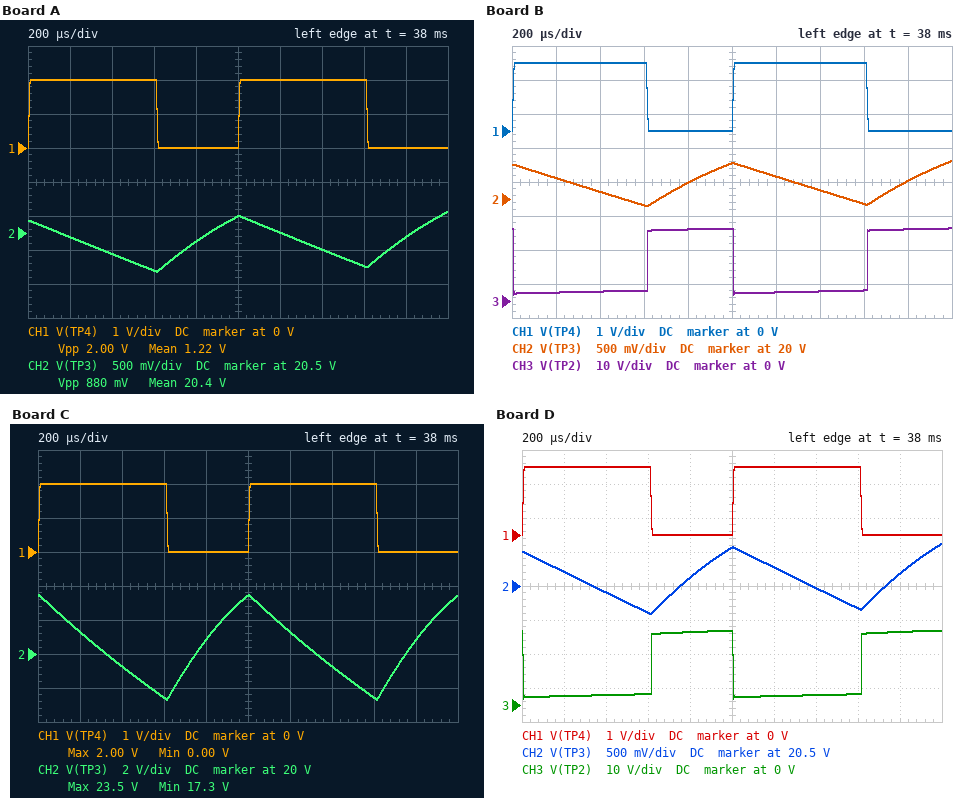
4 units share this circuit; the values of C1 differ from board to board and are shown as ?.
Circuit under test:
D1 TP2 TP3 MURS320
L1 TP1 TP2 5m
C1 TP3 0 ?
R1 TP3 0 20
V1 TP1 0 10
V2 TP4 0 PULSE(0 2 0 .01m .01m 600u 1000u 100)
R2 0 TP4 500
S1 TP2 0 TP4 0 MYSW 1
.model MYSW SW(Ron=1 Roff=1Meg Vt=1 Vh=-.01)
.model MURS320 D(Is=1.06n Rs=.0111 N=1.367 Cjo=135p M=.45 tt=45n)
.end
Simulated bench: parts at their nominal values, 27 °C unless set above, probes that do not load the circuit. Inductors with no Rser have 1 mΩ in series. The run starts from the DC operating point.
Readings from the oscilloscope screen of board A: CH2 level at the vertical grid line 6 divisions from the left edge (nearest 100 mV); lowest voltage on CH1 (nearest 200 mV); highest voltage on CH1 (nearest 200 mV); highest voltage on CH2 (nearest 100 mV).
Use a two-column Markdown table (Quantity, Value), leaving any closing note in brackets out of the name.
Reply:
| Quantity | Value |
|---|---|
| CH2 level at the vertical grid line 6 divisions from the left edge | 20.5 V |
| lowest voltage on CH1 | 0 V |
| highest voltage on CH1 | 2.0 V |
| highest voltage on CH2 | 20.8 V |
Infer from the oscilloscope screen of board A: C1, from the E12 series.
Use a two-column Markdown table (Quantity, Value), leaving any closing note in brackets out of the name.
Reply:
| Quantity | Value |
|---|---|
| C1, from the E12 series | 820 µF |
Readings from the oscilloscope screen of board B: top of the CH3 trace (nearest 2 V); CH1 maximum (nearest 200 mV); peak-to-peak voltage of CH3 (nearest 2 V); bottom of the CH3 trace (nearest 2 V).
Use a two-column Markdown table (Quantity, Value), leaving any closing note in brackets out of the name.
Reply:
| Quantity | Value |
|---|---|
| top of the CH3 trace | 22 V |
| CH1 maximum | 2.0 V |
| peak-to-peak voltage of CH3 | 20 V |
| bottom of the CH3 trace | 2 V |
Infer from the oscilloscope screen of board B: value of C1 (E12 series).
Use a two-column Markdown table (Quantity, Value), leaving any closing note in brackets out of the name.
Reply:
| Quantity | Value |
|---|---|
| value of C1 | 1 mF |
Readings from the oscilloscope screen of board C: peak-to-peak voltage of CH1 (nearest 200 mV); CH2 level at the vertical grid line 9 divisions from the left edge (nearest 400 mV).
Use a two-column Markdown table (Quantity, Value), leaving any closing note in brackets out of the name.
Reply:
| Quantity | Value |
|---|---|
| peak-to-peak voltage of CH1 | 2.0 V |
| CH2 level at the vertical grid line 9 divisions from the left edge | 20.8 V |
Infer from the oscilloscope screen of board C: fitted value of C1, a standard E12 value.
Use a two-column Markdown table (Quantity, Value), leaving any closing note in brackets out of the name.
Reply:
| Quantity | Value |
|---|---|
| fitted value of C1, a standard E12 value | 100 µF |
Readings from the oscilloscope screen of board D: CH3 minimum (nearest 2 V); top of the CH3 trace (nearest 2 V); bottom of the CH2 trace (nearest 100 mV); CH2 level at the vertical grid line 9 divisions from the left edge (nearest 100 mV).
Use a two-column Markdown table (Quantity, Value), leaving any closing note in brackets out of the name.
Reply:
| Quantity | Value |
|---|---|
| CH3 minimum | 2 V |
| top of the CH3 trace | 22 V |
| bottom of the CH2 trace | 20.1 V |
| CH2 level at the vertical grid line 9 divisions from the left edge | 20.7 V |
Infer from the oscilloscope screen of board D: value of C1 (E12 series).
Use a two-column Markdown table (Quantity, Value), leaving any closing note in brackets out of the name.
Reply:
| Quantity | Value |
|---|---|
| value of C1 | 680 µF |
